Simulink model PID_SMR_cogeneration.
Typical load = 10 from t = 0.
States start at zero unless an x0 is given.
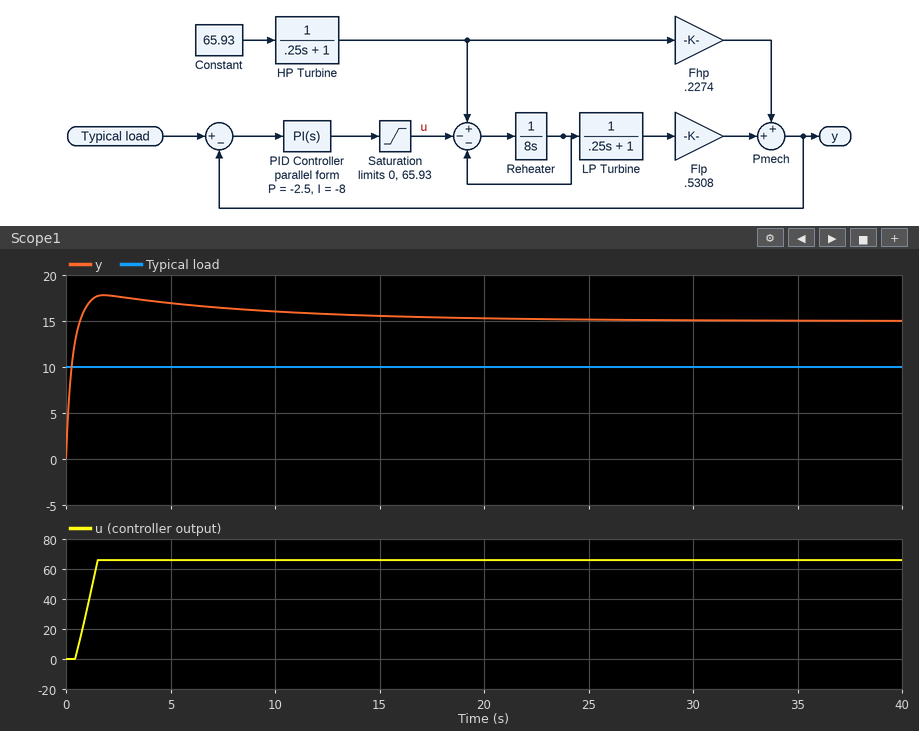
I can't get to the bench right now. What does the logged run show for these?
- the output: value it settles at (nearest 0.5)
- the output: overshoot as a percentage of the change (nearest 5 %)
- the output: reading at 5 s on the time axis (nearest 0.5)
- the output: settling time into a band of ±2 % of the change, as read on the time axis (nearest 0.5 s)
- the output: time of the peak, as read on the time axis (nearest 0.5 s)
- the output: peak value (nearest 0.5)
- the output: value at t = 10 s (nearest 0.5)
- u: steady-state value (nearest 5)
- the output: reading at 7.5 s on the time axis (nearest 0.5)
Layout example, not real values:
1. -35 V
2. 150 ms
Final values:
1. 15.0
2. 20 %
3. 17.0
4. 20.0 s
5. 2.0 s
6. 18.0
7. 16.0
8. 65
9. 16.5
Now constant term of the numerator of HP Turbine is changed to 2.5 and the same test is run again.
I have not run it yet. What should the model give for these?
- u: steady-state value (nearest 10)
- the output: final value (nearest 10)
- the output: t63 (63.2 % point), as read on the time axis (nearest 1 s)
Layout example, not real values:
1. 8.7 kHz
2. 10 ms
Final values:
1. 70
2. 90
3. 4 s
